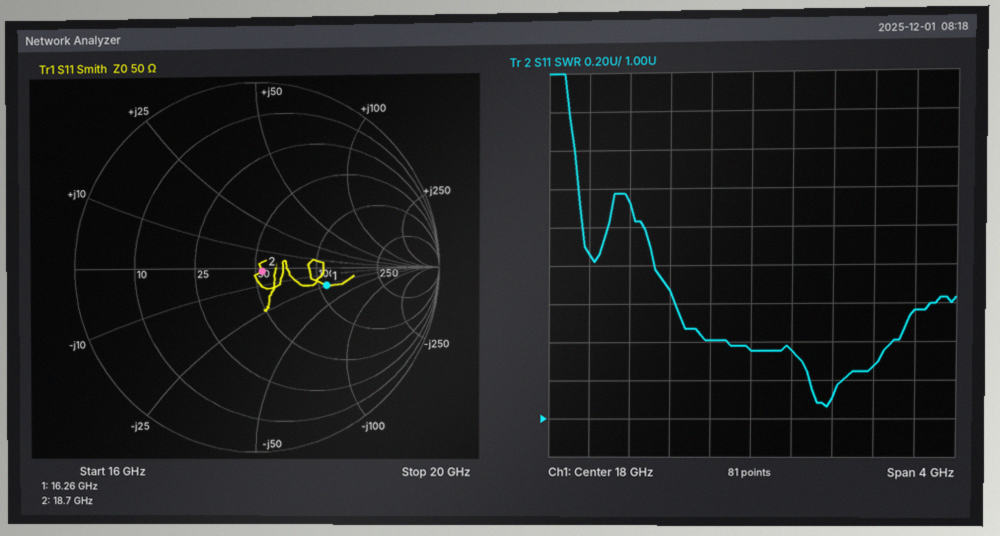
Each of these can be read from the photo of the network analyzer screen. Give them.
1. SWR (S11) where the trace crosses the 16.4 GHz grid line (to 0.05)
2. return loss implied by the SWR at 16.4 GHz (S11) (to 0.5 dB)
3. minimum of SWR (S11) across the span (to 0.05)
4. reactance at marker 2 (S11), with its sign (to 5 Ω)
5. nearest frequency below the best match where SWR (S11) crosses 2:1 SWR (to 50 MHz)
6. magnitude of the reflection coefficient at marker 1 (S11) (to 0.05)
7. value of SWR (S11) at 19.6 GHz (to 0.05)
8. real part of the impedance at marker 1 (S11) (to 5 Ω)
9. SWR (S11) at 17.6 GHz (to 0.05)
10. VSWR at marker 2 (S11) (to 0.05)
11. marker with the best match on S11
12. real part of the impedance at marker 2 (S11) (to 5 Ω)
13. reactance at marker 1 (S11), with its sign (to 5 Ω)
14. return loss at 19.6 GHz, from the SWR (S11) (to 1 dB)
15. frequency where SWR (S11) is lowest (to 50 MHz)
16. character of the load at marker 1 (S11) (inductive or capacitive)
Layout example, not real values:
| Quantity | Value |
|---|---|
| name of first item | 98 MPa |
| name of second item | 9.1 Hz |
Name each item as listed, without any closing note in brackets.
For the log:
| Quantity | Value |
|---|---|
| SWR (S11) where the trace crosses the 16.4 GHz grid line | 1.85 |
| return loss implied by the SWR at 16.4 GHz (S11) | 10.5 dB |
| minimum of SWR (S11) across the span | 1.05 |
| reactance at marker 2 (S11), with its sign | 0 Ω |
| nearest frequency below the best match where SWR (S11) crosses 2:1 SWR | 16.95 GHz |
| magnitude of the reflection coefficient at marker 1 (S11) | 0.40 |
| value of SWR (S11) at 19.6 GHz | 1.55 |
| real part of the impedance at marker 1 (S11) | 110 Ω |
| SWR (S11) at 17.6 GHz | 1.40 |
| VSWR at marker 2 (S11) | 1.10 |
| marker with the best match on S11 | marker 2 |
| real part of the impedance at marker 2 (S11) | 55 Ω |
| reactance at marker 1 (S11), with its sign | -25 Ω |
| return loss at 19.6 GHz, from the SWR (S11) | 13 dB |
| frequency where SWR (S11) is lowest | 18.75 GHz |
| character of the load at marker 1 (S11) | capacitive |
